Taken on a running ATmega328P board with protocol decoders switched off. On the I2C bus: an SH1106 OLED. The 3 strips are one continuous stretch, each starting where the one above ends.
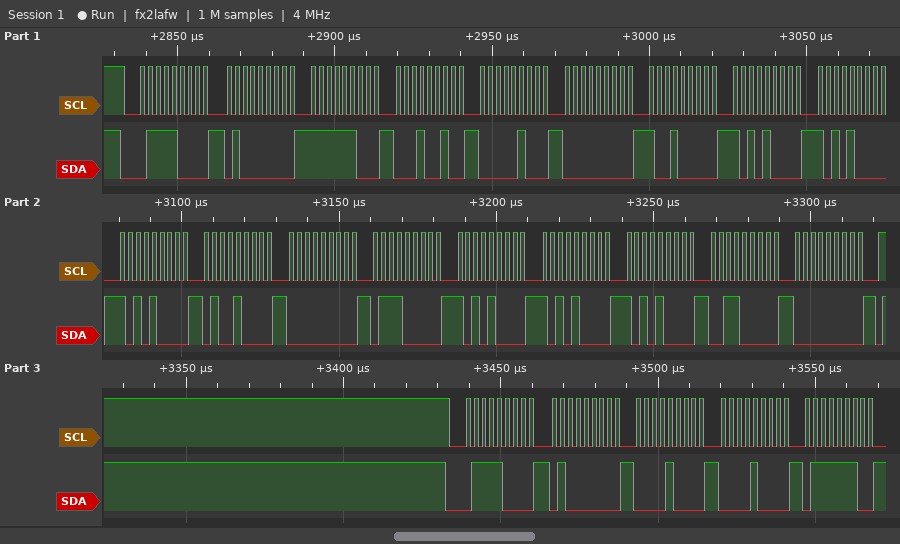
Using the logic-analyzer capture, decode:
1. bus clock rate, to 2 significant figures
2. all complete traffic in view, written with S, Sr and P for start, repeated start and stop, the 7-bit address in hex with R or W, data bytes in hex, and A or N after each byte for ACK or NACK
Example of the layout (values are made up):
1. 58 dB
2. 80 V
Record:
1. 400 kHz
2. S 3CW A 40 A FC A 12 A 04 A 00 A 90 A A8 A A8 A A8 A 48 A 00 A 70 A A8 A A8 A A8 A 30 A 00 A P S 3CW A 40 A 08 A 08 A 7E A
